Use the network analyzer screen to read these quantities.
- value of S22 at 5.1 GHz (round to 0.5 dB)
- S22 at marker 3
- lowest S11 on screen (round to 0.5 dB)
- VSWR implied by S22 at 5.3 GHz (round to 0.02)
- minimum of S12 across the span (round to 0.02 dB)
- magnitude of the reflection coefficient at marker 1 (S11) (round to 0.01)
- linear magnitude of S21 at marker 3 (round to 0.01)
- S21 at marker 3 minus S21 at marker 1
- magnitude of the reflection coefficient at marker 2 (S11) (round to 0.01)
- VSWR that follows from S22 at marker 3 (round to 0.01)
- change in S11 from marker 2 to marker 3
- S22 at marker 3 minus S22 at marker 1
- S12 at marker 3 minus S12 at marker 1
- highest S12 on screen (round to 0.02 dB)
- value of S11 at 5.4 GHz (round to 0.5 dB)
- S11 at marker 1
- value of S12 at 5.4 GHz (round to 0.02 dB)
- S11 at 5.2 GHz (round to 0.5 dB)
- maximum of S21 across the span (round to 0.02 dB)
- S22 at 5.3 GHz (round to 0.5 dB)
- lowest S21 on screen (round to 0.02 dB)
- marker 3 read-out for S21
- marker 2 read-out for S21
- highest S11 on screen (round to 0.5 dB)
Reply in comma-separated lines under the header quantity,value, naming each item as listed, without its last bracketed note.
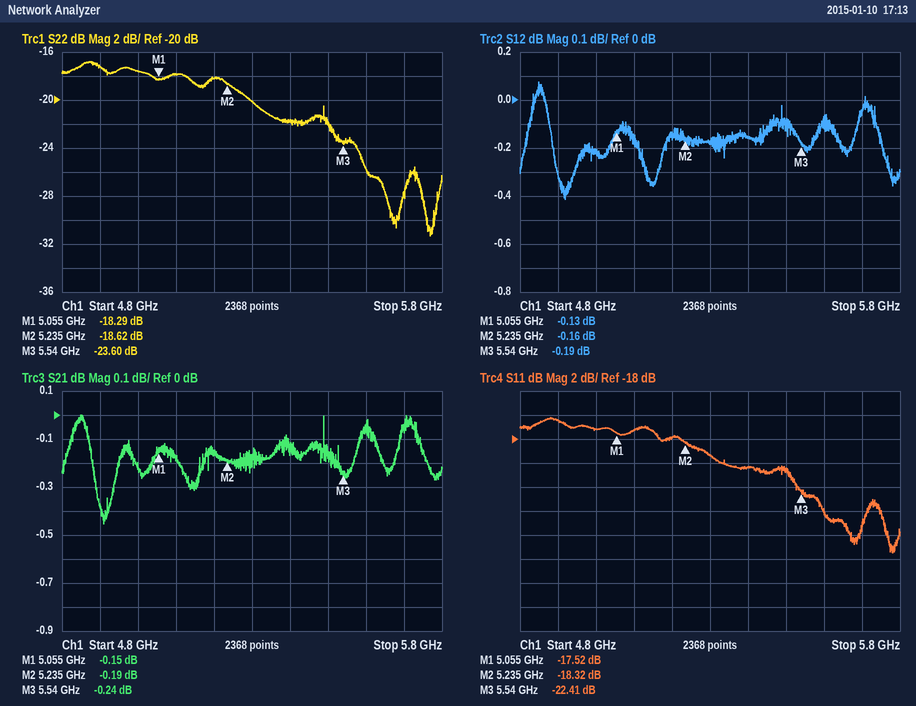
quantity,value
value of S22 at 5.1 GHz,-18.0 dB
S22 at marker 3,-23.60 dB
lowest S11 on screen,-27.5 dB
VSWR implied by S22 at 5.3 GHz,1.22
minimum of S12 across the span,-0.42 dB
magnitude of the reflection coefficient at marker 1 (S11),0.13
linear magnitude of S21 at marker 3,0.97
S21 at marker 3 minus S21 at marker 1,-0.09 dB
magnitude of the reflection coefficient at marker 2 (S11),0.12
VSWR that follows from S22 at marker 3,1.14
change in S11 from marker 2 to marker 3,-4.09 dB
S22 at marker 3 minus S22 at marker 1,-5.31 dB
S12 at marker 3 minus S12 at marker 1,-0.06 dB
highest S12 on screen,0.08 dB
value of S11 at 5.4 GHz,-20.5 dB
S11 at marker 1,-17.52 dB
value of S12 at 5.4 GHz,-0.16 dB
S11 at 5.2 GHz,-18.0 dB
maximum of S21 across the span,0.00 dB
S22 at 5.3 GHz,-20.0 dB
lowest S21 on screen,-0.46 dB
marker 3 read-out for S21,-0.24 dB
marker 2 read-out for S21,-0.19 dB
highest S11 on screen,-16.0 dB
